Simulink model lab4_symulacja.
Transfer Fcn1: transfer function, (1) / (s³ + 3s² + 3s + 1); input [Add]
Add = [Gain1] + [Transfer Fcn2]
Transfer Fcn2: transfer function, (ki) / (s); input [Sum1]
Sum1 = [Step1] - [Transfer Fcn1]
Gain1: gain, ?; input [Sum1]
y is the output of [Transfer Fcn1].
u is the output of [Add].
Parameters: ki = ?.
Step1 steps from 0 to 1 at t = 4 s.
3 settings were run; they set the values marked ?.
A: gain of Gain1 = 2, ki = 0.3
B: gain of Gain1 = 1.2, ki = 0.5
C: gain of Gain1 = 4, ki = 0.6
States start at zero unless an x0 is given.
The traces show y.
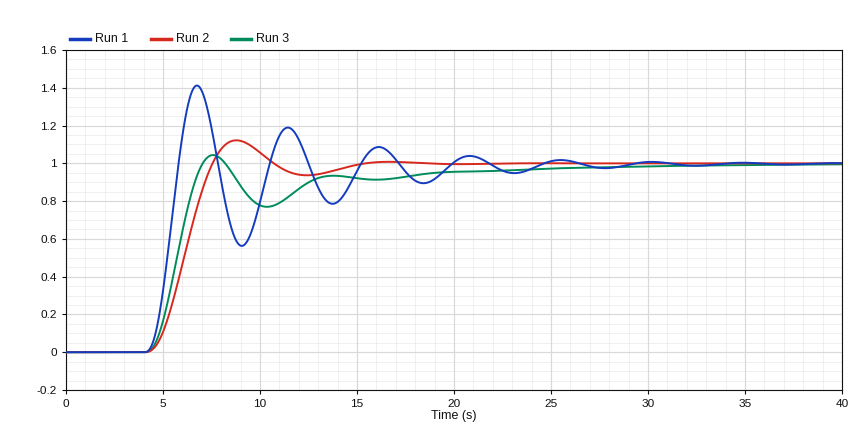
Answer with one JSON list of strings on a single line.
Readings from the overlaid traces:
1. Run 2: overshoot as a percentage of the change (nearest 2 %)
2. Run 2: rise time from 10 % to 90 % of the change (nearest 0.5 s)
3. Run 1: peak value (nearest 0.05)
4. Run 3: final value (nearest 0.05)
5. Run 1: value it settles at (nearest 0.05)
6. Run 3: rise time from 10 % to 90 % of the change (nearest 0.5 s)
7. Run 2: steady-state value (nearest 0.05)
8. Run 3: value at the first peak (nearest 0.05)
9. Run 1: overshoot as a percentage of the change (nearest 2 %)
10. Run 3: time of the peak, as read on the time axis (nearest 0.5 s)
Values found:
["12 %", "2.0 s", "1.40", "1.00", "1.00", "2.0 s", "1.00", "1.05", "42 %", "7.5 s"]
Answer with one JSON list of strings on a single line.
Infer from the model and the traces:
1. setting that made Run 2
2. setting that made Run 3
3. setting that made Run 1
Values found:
["B", "A", "C"]
